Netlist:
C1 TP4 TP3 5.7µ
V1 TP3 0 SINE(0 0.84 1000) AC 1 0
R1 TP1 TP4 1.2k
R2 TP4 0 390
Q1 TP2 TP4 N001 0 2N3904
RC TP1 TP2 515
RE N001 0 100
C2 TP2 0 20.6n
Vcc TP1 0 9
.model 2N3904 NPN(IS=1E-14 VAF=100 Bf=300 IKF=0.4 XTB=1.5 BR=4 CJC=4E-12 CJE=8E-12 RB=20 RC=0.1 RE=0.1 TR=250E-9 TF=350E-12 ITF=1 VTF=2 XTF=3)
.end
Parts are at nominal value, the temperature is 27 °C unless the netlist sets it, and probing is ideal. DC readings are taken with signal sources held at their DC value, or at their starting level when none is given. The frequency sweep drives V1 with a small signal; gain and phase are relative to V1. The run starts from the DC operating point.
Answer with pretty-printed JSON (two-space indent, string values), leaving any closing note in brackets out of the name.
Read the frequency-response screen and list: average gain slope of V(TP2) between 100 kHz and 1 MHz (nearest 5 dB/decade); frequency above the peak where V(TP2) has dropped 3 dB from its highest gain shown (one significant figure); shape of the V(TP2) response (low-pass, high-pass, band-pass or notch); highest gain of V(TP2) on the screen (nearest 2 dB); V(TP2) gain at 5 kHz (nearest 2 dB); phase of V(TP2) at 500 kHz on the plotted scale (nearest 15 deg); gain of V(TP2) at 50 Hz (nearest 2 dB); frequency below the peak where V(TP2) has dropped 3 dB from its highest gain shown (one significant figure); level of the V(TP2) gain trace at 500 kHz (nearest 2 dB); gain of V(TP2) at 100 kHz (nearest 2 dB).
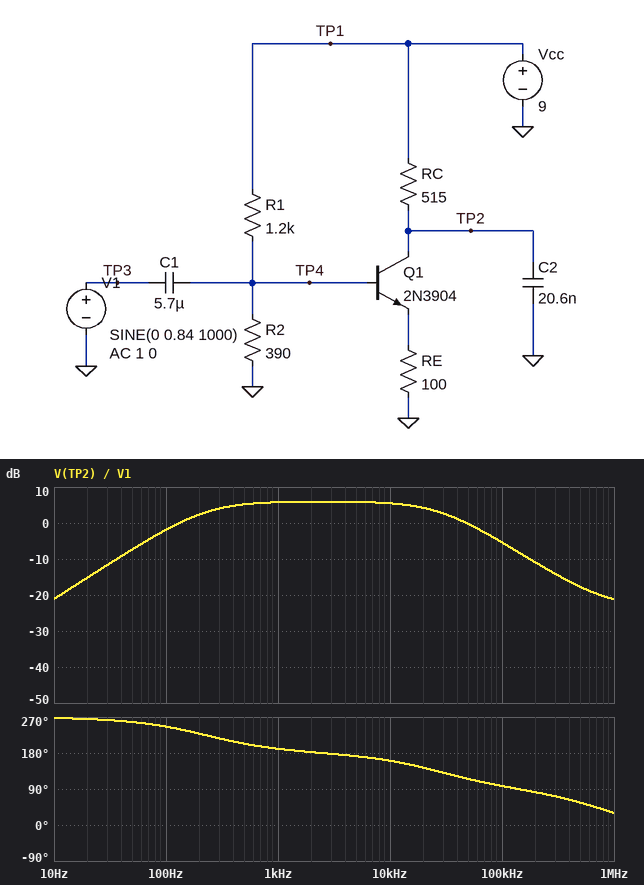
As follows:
{
  "average gain slope of V(TP2) between 100 kHz and 1 MHz": "-15 dB/decade",
  "frequency above the peak where V(TP2) has dropped 3 dB from its highest gain shown": "30 kHz",
  "shape of the V(TP2) response": "band-pass",
  "highest gain of V(TP2) on the screen": "6 dB",
  "V(TP2) gain at 5 kHz": "6 dB",
  "phase of V(TP2) at 500 kHz on the plotted scale": "60 deg",
  "gain of V(TP2) at 50 Hz": "-8 dB",
  "frequency below the peak where V(TP2) has dropped 3 dB from its highest gain shown": "200 Hz",
  "level of the V(TP2) gain trace at 500 kHz": "-18 dB",
  "gain of V(TP2) at 100 kHz": "-6 dB"
}
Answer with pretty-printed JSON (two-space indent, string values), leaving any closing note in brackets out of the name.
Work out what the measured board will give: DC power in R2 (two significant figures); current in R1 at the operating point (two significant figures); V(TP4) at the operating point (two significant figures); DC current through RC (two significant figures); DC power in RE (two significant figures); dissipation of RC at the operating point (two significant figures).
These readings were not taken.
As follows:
{
  "DC power in R2": "12 mW",
  "current in R1 at the operating point": "5.7 mA",
  "V(TP4) at the operating point": "2.2 V",
  "DC current through RC": "14 mA",
  "DC power in RE": "21 mW",
  "dissipation of RC at the operating point": "110 mW"
}
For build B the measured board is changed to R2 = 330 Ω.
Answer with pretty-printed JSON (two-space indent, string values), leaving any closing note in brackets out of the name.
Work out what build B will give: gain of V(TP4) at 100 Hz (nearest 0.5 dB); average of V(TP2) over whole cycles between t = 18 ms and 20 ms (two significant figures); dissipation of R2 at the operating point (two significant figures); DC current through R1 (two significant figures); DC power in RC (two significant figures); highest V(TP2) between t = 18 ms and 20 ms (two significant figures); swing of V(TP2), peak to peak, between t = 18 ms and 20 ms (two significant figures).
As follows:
{
  "gain of V(TP4) at 100 Hz": "-3.5 dB",
  "average of V(TP2) over whole cycles between t = 18 ms and 20 ms": "4.2 V",
  "dissipation of R2 at the operating point": "11 mW",
  "DC current through R1": "5.9 mA",
  "DC power in RC": "75 mW",
  "highest V(TP2) between t = 18 ms and 20 ms": "7.8 V",
  "swing of V(TP2), peak to peak, between t = 18 ms and 20 ms": "6.2 V"
}
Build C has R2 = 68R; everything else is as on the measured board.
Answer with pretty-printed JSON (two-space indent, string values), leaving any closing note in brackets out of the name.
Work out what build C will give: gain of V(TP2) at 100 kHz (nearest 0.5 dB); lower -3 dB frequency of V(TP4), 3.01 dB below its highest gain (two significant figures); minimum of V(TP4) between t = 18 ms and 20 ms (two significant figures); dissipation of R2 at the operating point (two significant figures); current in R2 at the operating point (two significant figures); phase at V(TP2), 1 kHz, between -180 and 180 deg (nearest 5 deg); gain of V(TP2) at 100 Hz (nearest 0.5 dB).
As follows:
{
  "gain of V(TP2) at 100 kHz": "-48.0 dB",
  "lower -3 dB frequency of V(TP4), 3.01 dB below its highest gain": "430 Hz",
  "minimum of V(TP4) between t = 18 ms and 20 ms": "-290 mV",
  "dissipation of R2 at the operating point": "3.4 mW",
  "current in R2 at the operating point": "7.1 mA",
  "phase at V(TP2), 1 kHz, between -180 and 180 deg": "-160 deg",
  "gain of V(TP2) at 100 Hz": "-44.5 dB"
}
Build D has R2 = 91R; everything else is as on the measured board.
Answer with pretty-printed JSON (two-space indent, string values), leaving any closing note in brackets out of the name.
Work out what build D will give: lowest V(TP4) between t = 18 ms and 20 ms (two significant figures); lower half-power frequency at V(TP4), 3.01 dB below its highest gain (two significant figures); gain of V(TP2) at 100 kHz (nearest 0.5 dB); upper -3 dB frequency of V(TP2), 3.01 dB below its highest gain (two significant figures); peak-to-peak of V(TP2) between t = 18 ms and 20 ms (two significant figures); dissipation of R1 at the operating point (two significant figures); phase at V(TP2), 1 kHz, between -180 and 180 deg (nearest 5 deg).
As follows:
{
  "lowest V(TP4) between t = 18 ms and 20 ms": "-160 mV",
  "lower half-power frequency at V(TP4), 3.01 dB below its highest gain": "330 Hz",
  "gain of V(TP2) at 100 kHz": "-9.5 dB",
  "upper -3 dB frequency of V(TP2), 3.01 dB below its highest gain": "16 kHz",
  "peak-to-peak of V(TP2) between t = 18 ms and 20 ms": "3.7 V",
  "dissipation of R1 at the operating point": "58 mW",
  "phase at V(TP2), 1 kHz, between -180 and 180 deg": "-165 deg"
}
